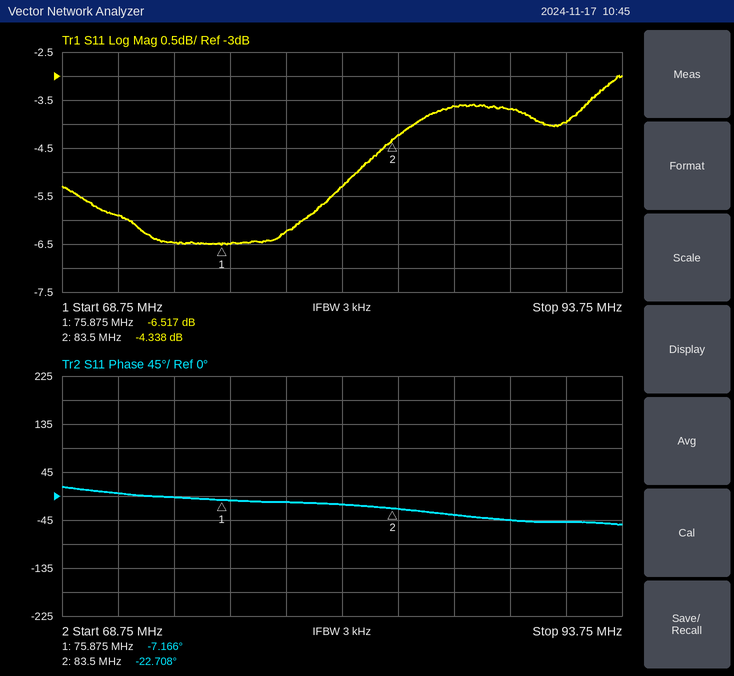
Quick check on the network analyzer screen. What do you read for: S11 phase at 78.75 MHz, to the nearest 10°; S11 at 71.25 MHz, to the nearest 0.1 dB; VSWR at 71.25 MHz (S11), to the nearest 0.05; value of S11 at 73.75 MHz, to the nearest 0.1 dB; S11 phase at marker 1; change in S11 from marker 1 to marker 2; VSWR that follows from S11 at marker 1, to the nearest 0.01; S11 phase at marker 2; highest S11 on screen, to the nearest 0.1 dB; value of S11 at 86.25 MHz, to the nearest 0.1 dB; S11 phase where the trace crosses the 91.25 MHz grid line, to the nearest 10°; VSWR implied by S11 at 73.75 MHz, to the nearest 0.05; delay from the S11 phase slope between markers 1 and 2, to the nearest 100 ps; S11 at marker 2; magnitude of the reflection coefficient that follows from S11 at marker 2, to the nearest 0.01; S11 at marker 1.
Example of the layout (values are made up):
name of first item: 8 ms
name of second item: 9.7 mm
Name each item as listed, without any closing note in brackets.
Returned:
S11 phase at 78.75 MHz, to the nearest 10°: -10°
S11 at 71.25 MHz, to the nearest 0.1 dB: -5.9 dB
VSWR at 71.25 MHz (S11), to the nearest 0.05: 3.05
value of S11 at 73.75 MHz, to the nearest 0.1 dB: -6.5 dB
S11 phase at marker 1: -7.166°
change in S11 from marker 1 to marker 2: 2.179 dB
VSWR that follows from S11 at marker 1, to the nearest 0.01: 2.79
S11 phase at marker 2: -22.708°
highest S11 on screen, to the nearest 0.1 dB: -3.0 dB
value of S11 at 86.25 MHz, to the nearest 0.1 dB: -3.6 dB
S11 phase where the trace crosses the 91.25 MHz grid line, to the nearest 10°: -50°
VSWR implied by S11 at 73.75 MHz, to the nearest 0.05: 2.80
delay from the S11 phase slope between markers 1 and 2, to the nearest 100 ps: 5.7 ns
S11 at marker 2: -4.338 dB
magnitude of the reflection coefficient that follows from S11 at marker 2, to the nearest 0.01: 0.61
S11 at marker 1: -6.517 dB
